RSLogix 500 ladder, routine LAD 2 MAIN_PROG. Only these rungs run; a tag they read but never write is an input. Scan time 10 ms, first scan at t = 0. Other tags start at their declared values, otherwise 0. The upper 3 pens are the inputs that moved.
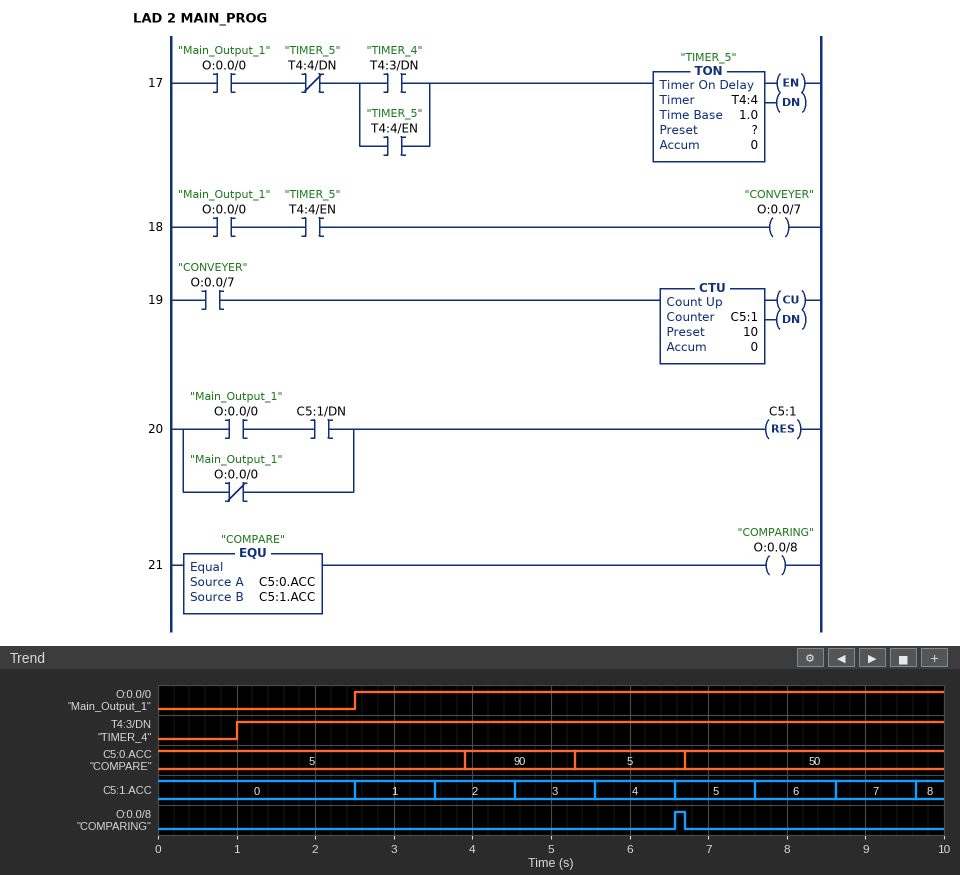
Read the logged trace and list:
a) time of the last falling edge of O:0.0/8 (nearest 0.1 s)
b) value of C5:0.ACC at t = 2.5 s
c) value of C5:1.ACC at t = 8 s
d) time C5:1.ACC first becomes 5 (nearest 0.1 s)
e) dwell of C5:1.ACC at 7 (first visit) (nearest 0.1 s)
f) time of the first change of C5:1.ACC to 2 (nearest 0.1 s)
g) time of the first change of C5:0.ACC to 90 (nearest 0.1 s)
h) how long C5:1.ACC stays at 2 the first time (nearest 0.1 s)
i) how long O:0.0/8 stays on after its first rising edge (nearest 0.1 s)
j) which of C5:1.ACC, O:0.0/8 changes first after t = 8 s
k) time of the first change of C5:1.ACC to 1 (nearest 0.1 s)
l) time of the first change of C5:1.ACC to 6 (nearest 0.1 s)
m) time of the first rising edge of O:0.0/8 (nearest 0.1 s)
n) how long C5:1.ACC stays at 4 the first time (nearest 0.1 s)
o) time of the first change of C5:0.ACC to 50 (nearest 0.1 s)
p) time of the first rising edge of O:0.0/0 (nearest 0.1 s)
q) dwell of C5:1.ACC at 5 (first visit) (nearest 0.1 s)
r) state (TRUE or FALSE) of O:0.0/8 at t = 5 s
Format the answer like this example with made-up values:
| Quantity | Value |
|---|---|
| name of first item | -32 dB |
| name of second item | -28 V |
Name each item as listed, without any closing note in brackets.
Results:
| Quantity | Value |
|---|---|
| time of the last falling edge of O:0.0/8 | 6.7 s |
| value of C5:0.ACC at t = 2.5 s | 5 |
| value of C5:1.ACC at t = 8 s | 6 |
| time C5:1.ACC first becomes 5 | 6.6 s |
| dwell of C5:1.ACC at 7 (first visit) | 1.0 s |
| time of the first change of C5:1.ACC to 2 | 3.5 s |
| time of the first change of C5:0.ACC to 90 | 3.9 s |
| how long C5:1.ACC stays at 2 the first time | 1.0 s |
| how long O:0.0/8 stays on after its first rising edge | 0.1 s |
| which of C5:1.ACC, O:0.0/8 changes first after t = 8 s | C5:1.ACC |
| time of the first change of C5:1.ACC to 1 | 2.5 s |
| time of the first change of C5:1.ACC to 6 | 7.6 s |
| time of the first rising edge of O:0.0/8 | 6.6 s |
| how long C5:1.ACC stays at 4 the first time | 1.0 s |
| time of the first change of C5:0.ACC to 50 | 6.7 s |
| time of the first rising edge of O:0.0/0 | 2.5 s |
| dwell of C5:1.ACC at 5 (first visit) | 1.0 s |
| state (TRUE or FALSE) of O:0.0/8 at t = 5 s | FALSE |
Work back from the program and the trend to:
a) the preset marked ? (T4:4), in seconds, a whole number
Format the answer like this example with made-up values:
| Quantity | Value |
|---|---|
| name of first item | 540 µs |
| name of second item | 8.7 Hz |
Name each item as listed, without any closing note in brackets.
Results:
| Quantity | Value |
|---|---|
| the preset marked ? (T4:4), in seconds, a whole number | 1 s |
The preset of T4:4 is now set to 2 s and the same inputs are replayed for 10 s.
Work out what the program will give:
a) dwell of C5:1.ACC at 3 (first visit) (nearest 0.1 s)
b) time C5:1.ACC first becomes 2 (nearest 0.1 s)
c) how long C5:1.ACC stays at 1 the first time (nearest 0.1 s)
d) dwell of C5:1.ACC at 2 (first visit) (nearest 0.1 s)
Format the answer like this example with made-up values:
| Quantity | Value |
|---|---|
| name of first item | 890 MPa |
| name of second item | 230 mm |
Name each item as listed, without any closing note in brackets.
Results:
| Quantity | Value |
|---|---|
| dwell of C5:1.ACC at 3 (first visit) | 2.0 s |
| time C5:1.ACC first becomes 2 | 4.5 s |
| how long C5:1.ACC stays at 1 the first time | 2.0 s |
| dwell of C5:1.ACC at 2 (first visit) | 2.0 s |
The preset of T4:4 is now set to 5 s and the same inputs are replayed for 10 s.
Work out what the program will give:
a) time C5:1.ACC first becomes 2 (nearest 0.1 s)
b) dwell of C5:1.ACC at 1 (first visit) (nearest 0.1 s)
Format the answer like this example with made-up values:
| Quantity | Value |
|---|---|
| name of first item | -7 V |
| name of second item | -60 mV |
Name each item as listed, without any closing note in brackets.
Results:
| Quantity | Value |
|---|---|
| time C5:1.ACC first becomes 2 | 7.5 s |
| dwell of C5:1.ACC at 1 (first visit) | 5.0 s |
